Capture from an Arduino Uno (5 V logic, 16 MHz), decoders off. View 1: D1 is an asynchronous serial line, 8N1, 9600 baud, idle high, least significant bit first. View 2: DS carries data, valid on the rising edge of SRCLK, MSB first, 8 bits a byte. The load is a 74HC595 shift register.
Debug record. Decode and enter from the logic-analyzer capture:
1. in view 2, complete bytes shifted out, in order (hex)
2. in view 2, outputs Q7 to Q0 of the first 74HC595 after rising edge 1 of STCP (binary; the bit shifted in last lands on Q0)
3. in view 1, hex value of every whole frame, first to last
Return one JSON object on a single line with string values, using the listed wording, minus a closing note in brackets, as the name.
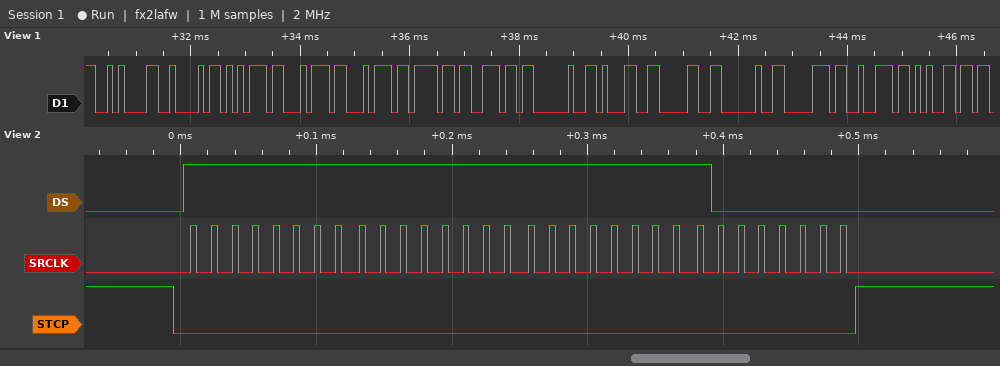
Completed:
{"in view 2, complete bytes shifted out, in order": "FF FF FF 80", "in view 2, outputs Q7 to Q0 of the first 74HC595 after rising edge 1 of STCP": "10000000", "in view 1, hex value of every whole frame, first to last": "0A 42 75 74 74 6F 6E 20 31 30 20 70 72 65"}
